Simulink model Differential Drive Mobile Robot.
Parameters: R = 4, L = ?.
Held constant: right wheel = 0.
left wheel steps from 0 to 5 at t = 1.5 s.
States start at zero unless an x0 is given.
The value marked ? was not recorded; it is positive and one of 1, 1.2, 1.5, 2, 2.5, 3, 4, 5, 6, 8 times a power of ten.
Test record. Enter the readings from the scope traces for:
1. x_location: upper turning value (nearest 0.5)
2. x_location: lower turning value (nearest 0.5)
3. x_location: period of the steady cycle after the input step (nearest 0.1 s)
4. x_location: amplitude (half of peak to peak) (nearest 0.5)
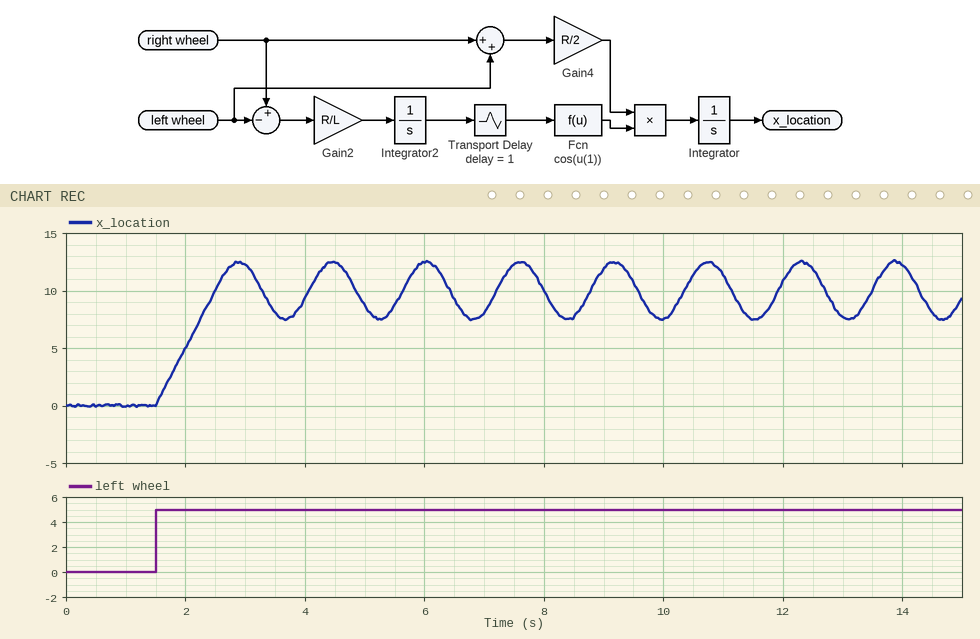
12.5
7.5
1.6 s
2.5
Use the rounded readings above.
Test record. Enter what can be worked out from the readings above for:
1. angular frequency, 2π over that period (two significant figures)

3.9 rad/s
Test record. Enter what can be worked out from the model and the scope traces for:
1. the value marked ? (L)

5
